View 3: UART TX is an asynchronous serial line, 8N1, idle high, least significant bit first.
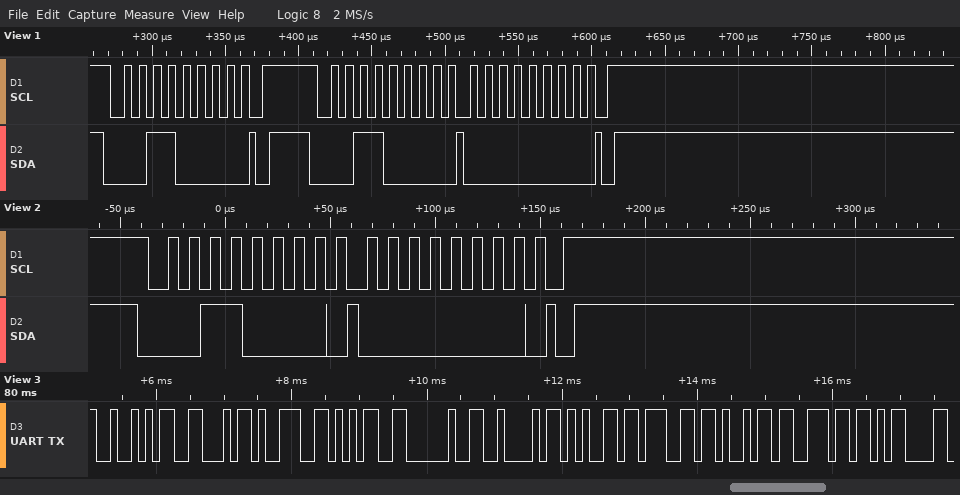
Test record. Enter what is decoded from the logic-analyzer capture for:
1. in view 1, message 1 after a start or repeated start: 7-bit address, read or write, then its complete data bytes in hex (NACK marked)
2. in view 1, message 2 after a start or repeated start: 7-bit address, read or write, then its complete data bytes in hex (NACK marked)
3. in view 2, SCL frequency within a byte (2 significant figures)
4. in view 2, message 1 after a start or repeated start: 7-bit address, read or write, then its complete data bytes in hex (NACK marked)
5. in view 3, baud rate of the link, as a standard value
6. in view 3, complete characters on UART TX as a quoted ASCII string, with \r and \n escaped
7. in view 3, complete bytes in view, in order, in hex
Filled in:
0x18 write
0x18 write: 00
100 kHz
0x18 write: 00
9600 baud
"RF95 Begin\r"
52 46 39 35 20 42 65 67 69 6E 0D
